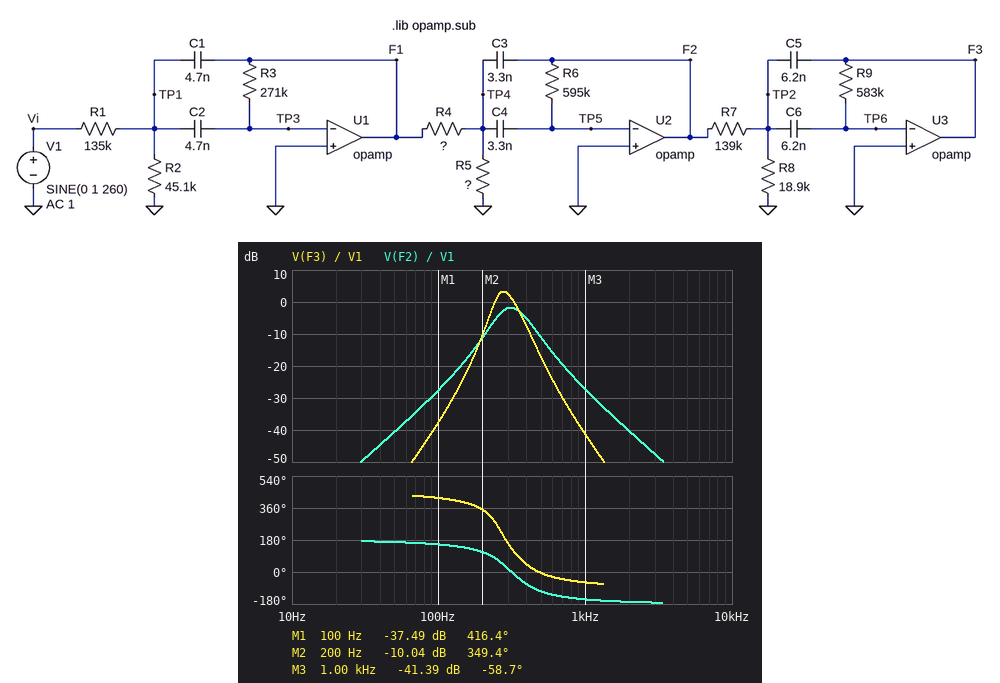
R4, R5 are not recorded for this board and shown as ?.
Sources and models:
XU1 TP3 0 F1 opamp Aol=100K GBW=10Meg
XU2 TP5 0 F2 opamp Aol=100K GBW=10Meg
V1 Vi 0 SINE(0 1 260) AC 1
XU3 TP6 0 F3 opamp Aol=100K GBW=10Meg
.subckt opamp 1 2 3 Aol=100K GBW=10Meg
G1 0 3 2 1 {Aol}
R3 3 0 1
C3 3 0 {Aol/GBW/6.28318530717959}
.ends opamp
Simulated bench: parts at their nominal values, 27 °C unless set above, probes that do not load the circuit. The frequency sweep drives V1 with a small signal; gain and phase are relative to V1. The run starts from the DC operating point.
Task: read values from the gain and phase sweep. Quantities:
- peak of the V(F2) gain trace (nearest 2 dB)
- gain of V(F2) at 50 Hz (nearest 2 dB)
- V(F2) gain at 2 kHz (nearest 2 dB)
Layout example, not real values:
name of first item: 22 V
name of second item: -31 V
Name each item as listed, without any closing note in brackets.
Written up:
peak of the V(F2) gain trace: -2 dB
gain of V(F2) at 50 Hz: -40 dB
V(F2) gain at 2 kHz: -40 dB
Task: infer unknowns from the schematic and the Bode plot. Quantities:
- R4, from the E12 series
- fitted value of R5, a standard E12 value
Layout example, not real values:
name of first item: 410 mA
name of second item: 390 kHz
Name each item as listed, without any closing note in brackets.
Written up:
R4, from the E12 series: 330 kΩ
fitted value of R5, a standard E12 value: 56 kΩ
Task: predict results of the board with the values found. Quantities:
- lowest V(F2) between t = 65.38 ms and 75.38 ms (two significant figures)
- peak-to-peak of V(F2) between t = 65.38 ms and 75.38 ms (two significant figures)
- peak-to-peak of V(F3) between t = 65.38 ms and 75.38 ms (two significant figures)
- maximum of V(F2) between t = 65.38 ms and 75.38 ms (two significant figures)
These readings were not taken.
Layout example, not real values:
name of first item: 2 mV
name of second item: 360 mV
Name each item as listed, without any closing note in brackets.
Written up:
lowest V(F2) between t = 65.38 ms and 75.38 ms: -640 mV
peak-to-peak of V(F2) between t = 65.38 ms and 75.38 ms: 1.3 V
peak-to-peak of V(F3) between t = 65.38 ms and 75.38 ms: 2.7 V
maximum of V(F2) between t = 65.38 ms and 75.38 ms: 640 mV
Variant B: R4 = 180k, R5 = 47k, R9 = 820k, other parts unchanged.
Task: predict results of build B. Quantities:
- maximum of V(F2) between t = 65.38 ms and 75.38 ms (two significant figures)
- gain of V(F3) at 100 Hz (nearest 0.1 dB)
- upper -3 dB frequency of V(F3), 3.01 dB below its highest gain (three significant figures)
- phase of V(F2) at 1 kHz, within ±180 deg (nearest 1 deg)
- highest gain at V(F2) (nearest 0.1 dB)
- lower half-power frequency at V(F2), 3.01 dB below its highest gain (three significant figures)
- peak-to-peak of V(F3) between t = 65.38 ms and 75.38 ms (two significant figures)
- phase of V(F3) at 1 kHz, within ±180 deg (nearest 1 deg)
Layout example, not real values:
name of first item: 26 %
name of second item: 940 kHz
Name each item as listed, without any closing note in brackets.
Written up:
maximum of V(F2) between t = 65.38 ms and 75.38 ms: 930 mV
gain of V(F3) at 100 Hz: -31.0 dB
upper -3 dB frequency of V(F3), 3.01 dB below its highest gain: 356 Hz
phase of V(F2) at 1 kHz, within ±180 deg: -154 deg
highest gain at V(F2): 4.2 dB
lower half-power frequency at V(F2), 3.01 dB below its highest gain: 277 Hz
peak-to-peak of V(F3) between t = 65.38 ms and 75.38 ms: 3.5 V
phase of V(F3) at 1 kHz, within ±180 deg: -60 deg
